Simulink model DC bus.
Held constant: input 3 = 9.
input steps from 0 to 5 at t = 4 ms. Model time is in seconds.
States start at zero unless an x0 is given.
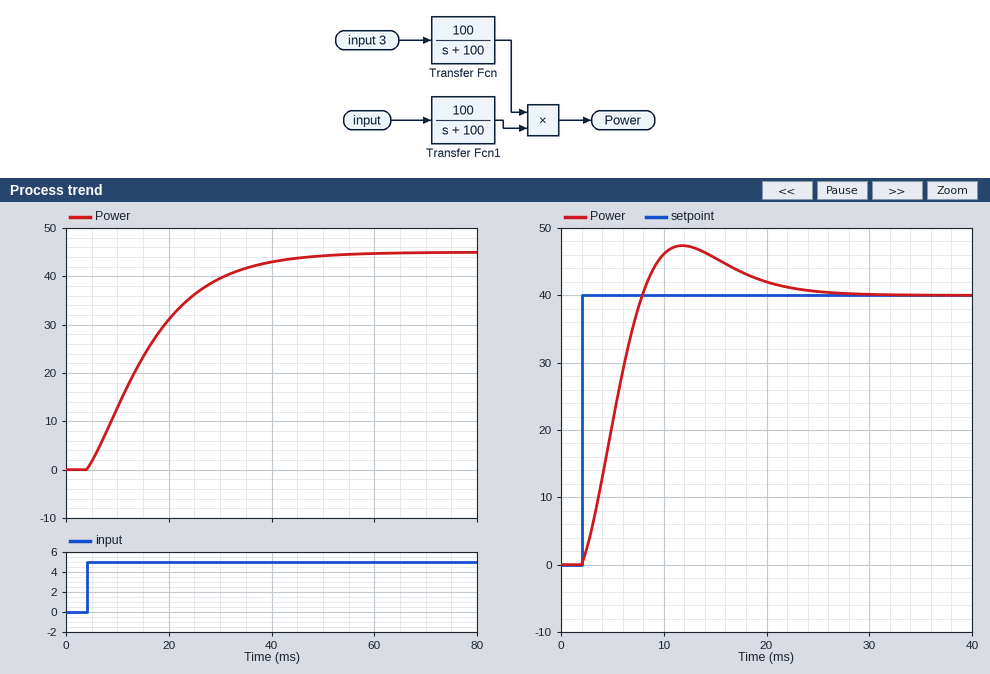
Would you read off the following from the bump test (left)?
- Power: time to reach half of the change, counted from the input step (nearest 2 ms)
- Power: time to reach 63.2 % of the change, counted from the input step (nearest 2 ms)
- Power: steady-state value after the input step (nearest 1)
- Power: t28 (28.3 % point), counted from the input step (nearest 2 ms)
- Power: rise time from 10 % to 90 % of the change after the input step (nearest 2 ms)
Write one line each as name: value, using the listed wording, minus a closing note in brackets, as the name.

Power: time to reach half of the change, counted from the input step: 10 ms
Power: time to reach 63.2 % of the change, counted from the input step: 14 ms
Power: steady-state value after the input step: 45
Power: t28 (28.3 % point), counted from the input step: 6 ms
Power: rise time from 10 % to 90 % of the change after the input step: 26 ms
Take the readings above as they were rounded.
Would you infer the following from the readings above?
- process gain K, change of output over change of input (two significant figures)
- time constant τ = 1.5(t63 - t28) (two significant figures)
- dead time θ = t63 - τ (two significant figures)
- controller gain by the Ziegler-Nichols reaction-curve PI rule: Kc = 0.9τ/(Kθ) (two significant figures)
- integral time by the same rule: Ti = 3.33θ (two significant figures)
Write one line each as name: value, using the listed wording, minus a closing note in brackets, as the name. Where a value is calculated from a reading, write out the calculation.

process gain K, change of output over change of input: (45 - 0) / 5 = 9.0
time constant τ = 1.5(t63 - t28): 1.5 × (14 - 6) = 12 ms
dead time θ = t63 - τ: 14 - 12 = 2.0 ms
controller gain by the Ziegler-Nichols reaction-curve PI rule: Kc = 0.9τ/(Kθ): 0.9 × 12 / (9 × 2) = 0.60
integral time by the same rule: Ti = 3.33θ: 3.33 × 2 = 6.7 ms
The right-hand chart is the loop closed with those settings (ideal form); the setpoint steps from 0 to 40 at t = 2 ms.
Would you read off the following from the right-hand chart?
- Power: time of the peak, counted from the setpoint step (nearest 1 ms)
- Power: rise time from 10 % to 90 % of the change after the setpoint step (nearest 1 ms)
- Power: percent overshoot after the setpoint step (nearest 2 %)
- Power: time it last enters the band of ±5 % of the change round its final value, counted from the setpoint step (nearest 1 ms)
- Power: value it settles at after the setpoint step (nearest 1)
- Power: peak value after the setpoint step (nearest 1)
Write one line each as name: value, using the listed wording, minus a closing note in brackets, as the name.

Power: time of the peak, counted from the setpoint step: 10 ms
Power: rise time from 10 % to 90 % of the change after the setpoint step: 4 ms
Power: percent overshoot after the setpoint step: 18 %
Power: time it last enters the band of ±5 % of the change round its final value, counted from the setpoint step: 18 ms
Power: value it settles at after the setpoint step: 40
Power: peak value after the setpoint step: 47
